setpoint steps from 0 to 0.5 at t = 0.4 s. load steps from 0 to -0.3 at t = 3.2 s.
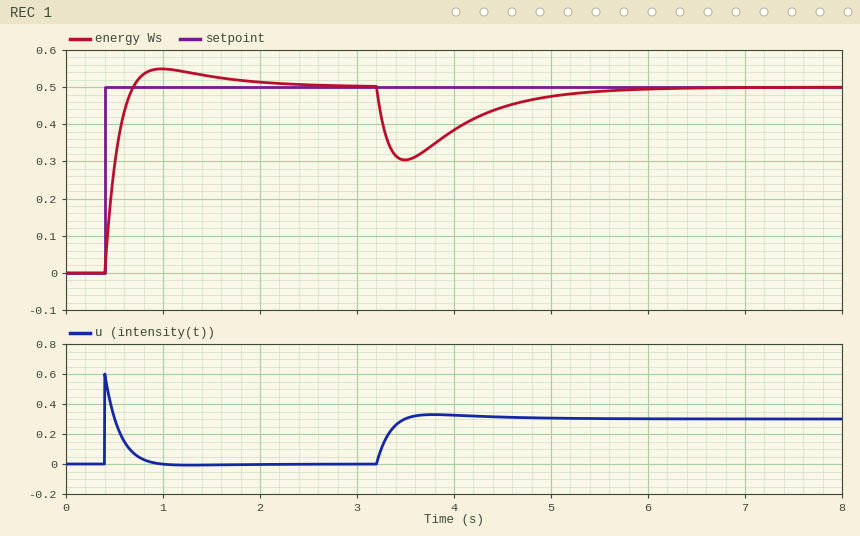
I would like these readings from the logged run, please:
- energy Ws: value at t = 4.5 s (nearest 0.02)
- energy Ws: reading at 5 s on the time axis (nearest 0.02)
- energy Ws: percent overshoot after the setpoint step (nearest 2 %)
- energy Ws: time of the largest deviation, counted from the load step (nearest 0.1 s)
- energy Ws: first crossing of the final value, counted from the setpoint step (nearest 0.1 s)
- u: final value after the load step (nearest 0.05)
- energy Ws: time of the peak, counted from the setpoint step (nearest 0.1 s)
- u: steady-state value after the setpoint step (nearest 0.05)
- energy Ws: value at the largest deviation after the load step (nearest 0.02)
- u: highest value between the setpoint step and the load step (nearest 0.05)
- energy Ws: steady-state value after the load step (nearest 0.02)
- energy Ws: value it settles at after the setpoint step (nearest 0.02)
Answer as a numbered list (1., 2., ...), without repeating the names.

1. 0.44
2. 0.48
3. 10 %
4. 0.3 s
5. 0.3 s
6. 0.30
7. 0.6 s
8. 0.00
9. 0.30
10. 0.60
11. 0.50
12. 0.50
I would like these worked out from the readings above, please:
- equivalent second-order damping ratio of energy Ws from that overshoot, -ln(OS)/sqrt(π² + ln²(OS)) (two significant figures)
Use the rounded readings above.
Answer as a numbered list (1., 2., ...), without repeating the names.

1. 0.59
